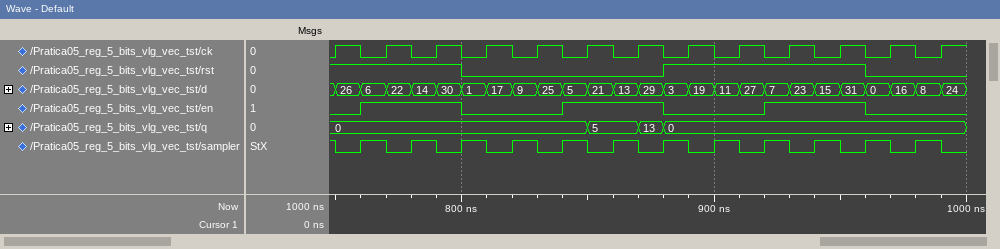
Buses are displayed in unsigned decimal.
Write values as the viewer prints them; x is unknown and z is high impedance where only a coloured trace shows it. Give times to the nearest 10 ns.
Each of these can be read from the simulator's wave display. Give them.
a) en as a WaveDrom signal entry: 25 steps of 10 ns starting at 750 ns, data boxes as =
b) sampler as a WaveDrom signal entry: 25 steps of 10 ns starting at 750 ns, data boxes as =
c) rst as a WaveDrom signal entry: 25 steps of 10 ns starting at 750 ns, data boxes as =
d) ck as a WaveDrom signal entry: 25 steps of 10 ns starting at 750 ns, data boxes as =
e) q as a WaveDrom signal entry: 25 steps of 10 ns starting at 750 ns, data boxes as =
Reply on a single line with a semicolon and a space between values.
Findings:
{name: 'en', wave: '01...0...1...0...1...0...'}; {name: 'sampler', wave: '0101010101010101010101010'}; {name: 'rst', wave: '1....0.......1.......0...'}; {name: 'ck', wave: '1010101010101010101010101'}; {name: 'q', wave: '=.........=.==...........', data: '0 5 13 0'}
